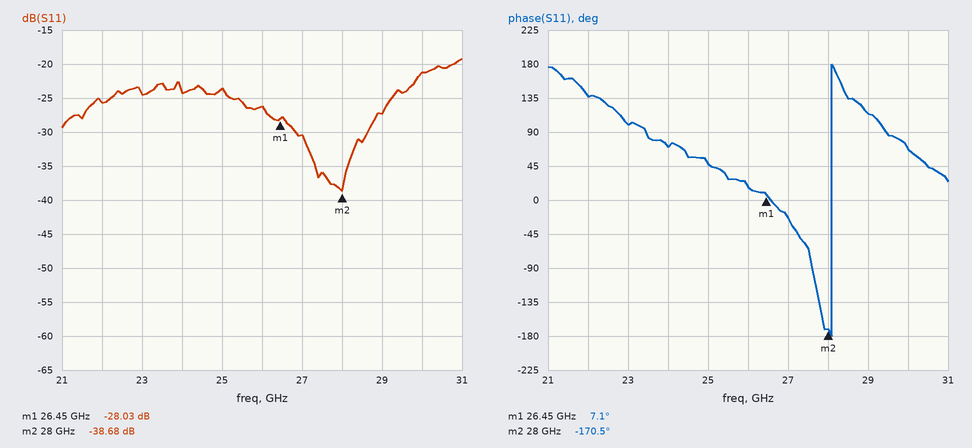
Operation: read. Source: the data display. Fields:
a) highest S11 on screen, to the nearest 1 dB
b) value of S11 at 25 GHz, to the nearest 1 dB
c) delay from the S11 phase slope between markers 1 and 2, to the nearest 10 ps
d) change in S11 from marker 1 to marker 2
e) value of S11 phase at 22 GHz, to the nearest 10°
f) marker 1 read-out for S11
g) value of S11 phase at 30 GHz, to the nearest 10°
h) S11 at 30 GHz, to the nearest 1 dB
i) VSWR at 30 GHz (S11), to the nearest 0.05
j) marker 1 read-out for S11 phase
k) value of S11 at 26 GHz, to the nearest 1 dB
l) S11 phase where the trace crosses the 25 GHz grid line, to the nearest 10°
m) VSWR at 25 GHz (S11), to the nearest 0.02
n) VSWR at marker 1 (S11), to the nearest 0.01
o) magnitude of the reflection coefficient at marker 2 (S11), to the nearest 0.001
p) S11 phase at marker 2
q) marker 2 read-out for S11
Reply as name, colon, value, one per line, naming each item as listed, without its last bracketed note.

highest S11 on screen, to the nearest 1 dB: -19 dB
value of S11 at 25 GHz, to the nearest 1 dB: -24 dB
delay from the S11 phase slope between markers 1 and 2, to the nearest 10 ps: 320 ps
change in S11 from marker 1 to marker 2: -10.65 dB
value of S11 phase at 22 GHz, to the nearest 10°: 140°
marker 1 read-out for S11: -28.03 dB
value of S11 phase at 30 GHz, to the nearest 10°: 70°
S11 at 30 GHz, to the nearest 1 dB: -21 dB
VSWR at 30 GHz (S11), to the nearest 0.05: 1.20
marker 1 read-out for S11 phase: 7.1°
value of S11 at 26 GHz, to the nearest 1 dB: -26 dB
S11 phase where the trace crosses the 25 GHz grid line, to the nearest 10°: 50°
VSWR at 25 GHz (S11), to the nearest 0.02: 1.14
VSWR at marker 1 (S11), to the nearest 0.01: 1.08
magnitude of the reflection coefficient at marker 2 (S11), to the nearest 0.001: 0.012
S11 phase at marker 2: -170.5°
marker 2 read-out for S11: -38.68 dB
